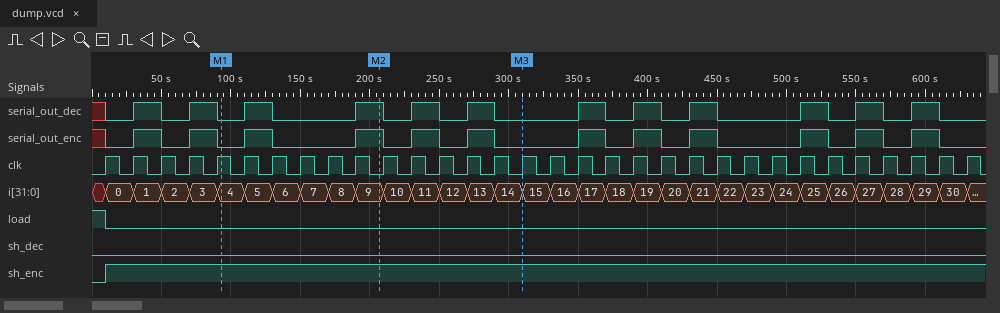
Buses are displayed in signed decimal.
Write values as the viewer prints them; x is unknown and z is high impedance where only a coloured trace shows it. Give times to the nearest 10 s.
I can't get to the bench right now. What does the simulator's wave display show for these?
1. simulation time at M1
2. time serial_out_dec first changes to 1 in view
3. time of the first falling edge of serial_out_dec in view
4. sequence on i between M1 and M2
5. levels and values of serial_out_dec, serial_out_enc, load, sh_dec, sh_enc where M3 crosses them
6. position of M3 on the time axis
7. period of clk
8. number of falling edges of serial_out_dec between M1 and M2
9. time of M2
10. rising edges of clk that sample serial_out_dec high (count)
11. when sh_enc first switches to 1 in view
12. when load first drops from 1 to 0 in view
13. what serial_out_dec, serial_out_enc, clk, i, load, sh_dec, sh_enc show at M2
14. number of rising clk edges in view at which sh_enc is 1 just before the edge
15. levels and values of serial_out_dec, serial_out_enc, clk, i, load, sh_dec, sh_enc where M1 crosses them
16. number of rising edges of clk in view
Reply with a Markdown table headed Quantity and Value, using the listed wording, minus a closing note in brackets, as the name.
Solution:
| Quantity | Value |
|---|---|
| simulation time at M1 | 90 s |
| time serial_out_dec first changes to 1 in view | 30 s |
| time of the first falling edge of serial_out_dec in view | 50 s |
| sequence on i between M1 and M2 | 4, 5, 6, 7, 8, 9 |
| levels and values of serial_out_dec, serial_out_enc, load, sh_dec, sh_enc where M3 crosses them | serial_out_dec=0, serial_out_enc=0, load=0, sh_dec=0, sh_enc=1 |
| position of M3 on the time axis | 310 s |
| period of clk | 20 s |
| number of falling edges of serial_out_dec between M1 and M2 | 1 |
| time of M2 | 210 s |
| rising edges of clk that sample serial_out_dec high | 12 |
| when sh_enc first switches to 1 in view | 10 s |
| when load first drops from 1 to 0 in view | 10 s |
| what serial_out_dec, serial_out_enc, clk, i, load, sh_dec, sh_enc show at M2 | serial_out_dec=1, serial_out_enc=1, clk=0, i=9, load=0, sh_dec=0, sh_enc=1 |
| number of rising clk edges in view at which sh_enc is 1 just before the edge | 31 |
| levels and values of serial_out_dec, serial_out_enc, clk, i, load, sh_dec, sh_enc where M1 crosses them | serial_out_dec=0, serial_out_enc=0, clk=1, i=4, load=0, sh_dec=0, sh_enc=1 |
| number of rising edges of clk in view | 32 |
